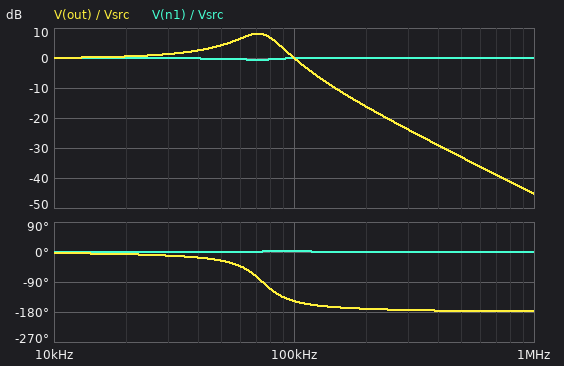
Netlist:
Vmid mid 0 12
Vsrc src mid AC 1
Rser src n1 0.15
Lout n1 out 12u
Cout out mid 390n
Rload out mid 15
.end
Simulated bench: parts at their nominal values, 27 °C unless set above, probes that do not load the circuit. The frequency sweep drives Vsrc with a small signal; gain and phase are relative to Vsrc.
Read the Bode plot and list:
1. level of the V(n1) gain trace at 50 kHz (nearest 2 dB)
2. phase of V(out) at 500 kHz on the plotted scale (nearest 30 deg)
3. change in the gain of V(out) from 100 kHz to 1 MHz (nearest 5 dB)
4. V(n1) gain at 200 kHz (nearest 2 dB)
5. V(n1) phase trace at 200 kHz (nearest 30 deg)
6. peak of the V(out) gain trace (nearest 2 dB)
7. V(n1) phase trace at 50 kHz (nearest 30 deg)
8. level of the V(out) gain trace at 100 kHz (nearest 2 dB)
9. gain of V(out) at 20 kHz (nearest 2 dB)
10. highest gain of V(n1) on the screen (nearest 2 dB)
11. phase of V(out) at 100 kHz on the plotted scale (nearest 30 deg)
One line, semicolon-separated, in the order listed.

0 dB; -180 deg; -45 dB; 0 dB; 0 deg; 8 dB; 0 deg; 0 dB; 0 dB; 0 dB; -150 deg
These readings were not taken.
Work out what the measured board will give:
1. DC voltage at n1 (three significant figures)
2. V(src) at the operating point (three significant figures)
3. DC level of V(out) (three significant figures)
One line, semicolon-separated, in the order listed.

12.0 V; 12.0 V; 12.0 V
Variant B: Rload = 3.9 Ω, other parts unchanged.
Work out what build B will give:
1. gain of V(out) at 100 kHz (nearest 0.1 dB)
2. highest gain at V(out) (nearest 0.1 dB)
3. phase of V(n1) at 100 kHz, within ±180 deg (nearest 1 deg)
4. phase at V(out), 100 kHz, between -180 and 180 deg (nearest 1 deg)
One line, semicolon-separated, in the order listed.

-6.6 dB; -0.3 dB; 1 deg; -112 deg
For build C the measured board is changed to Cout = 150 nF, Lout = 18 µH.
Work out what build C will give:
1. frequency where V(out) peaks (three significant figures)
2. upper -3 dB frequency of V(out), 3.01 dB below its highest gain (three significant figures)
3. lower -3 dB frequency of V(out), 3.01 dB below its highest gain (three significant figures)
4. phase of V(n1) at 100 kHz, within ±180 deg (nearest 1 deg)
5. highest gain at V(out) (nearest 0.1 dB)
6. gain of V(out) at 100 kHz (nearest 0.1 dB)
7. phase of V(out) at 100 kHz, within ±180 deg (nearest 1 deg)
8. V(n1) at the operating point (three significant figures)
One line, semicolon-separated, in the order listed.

82.9 kHz; 116 kHz; 19.0 kHz; 1 deg; 3.2 dB; 2.3 dB; -94 deg; 12.0 V
